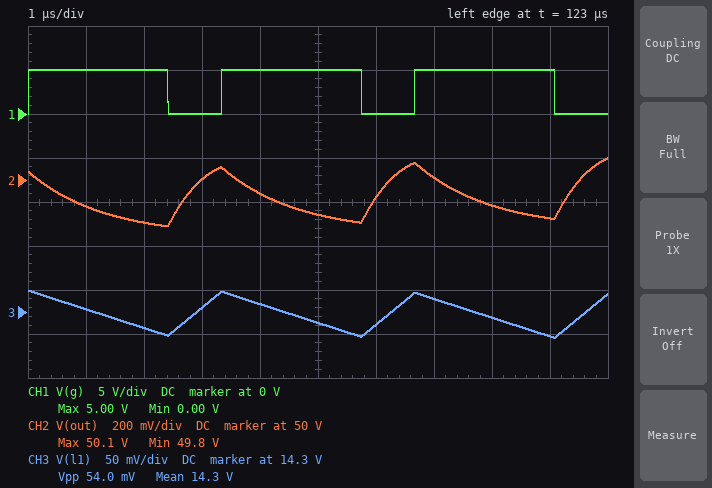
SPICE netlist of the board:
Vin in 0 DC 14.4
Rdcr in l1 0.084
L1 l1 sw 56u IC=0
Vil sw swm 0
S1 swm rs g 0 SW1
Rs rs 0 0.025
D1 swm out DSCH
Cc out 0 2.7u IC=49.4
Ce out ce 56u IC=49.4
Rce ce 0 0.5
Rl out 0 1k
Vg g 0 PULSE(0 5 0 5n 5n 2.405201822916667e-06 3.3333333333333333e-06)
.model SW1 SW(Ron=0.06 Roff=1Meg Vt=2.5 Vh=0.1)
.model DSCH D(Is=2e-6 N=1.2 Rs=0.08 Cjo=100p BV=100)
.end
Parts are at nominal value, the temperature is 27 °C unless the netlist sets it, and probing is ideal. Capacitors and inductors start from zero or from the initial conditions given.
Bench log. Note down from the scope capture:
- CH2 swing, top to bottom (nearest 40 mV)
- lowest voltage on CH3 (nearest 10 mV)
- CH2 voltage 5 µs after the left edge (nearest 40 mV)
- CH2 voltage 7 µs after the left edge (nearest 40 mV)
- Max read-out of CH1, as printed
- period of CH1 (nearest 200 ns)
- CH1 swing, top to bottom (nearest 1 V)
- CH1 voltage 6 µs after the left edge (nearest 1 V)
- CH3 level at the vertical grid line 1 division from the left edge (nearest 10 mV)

320 mV
14.27 V
49.84 V
50.00 V
5.00 V
3.4 µs
5 V
0 V
14.30 V
